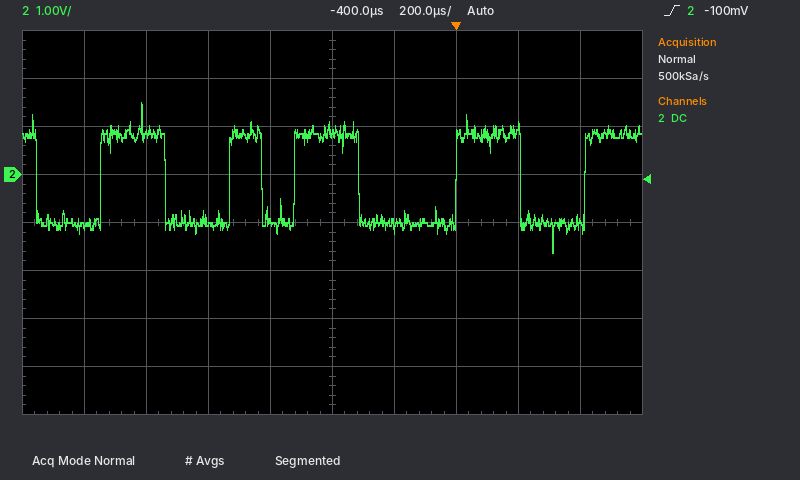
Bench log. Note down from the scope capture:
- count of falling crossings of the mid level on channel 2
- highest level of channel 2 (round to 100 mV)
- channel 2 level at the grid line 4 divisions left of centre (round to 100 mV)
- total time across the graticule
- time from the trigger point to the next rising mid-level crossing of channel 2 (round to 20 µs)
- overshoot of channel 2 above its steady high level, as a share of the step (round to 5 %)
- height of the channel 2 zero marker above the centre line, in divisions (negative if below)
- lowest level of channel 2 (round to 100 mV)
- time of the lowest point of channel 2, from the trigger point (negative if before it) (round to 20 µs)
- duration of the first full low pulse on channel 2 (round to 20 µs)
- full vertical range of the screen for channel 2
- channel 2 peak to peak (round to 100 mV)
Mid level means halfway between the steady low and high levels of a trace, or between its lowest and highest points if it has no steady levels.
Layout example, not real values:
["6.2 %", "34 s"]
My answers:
["5", "1.5 V", "-1.1 V", "2 ms", "420 µs", "35 %", "+1.0 div", "-1.6 V", "+320 µs", "200 µs", "8 V", "3.1 V"]
